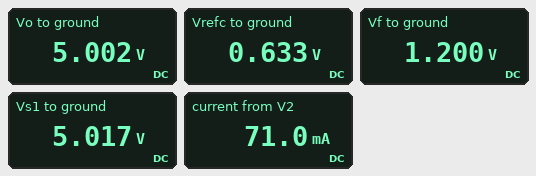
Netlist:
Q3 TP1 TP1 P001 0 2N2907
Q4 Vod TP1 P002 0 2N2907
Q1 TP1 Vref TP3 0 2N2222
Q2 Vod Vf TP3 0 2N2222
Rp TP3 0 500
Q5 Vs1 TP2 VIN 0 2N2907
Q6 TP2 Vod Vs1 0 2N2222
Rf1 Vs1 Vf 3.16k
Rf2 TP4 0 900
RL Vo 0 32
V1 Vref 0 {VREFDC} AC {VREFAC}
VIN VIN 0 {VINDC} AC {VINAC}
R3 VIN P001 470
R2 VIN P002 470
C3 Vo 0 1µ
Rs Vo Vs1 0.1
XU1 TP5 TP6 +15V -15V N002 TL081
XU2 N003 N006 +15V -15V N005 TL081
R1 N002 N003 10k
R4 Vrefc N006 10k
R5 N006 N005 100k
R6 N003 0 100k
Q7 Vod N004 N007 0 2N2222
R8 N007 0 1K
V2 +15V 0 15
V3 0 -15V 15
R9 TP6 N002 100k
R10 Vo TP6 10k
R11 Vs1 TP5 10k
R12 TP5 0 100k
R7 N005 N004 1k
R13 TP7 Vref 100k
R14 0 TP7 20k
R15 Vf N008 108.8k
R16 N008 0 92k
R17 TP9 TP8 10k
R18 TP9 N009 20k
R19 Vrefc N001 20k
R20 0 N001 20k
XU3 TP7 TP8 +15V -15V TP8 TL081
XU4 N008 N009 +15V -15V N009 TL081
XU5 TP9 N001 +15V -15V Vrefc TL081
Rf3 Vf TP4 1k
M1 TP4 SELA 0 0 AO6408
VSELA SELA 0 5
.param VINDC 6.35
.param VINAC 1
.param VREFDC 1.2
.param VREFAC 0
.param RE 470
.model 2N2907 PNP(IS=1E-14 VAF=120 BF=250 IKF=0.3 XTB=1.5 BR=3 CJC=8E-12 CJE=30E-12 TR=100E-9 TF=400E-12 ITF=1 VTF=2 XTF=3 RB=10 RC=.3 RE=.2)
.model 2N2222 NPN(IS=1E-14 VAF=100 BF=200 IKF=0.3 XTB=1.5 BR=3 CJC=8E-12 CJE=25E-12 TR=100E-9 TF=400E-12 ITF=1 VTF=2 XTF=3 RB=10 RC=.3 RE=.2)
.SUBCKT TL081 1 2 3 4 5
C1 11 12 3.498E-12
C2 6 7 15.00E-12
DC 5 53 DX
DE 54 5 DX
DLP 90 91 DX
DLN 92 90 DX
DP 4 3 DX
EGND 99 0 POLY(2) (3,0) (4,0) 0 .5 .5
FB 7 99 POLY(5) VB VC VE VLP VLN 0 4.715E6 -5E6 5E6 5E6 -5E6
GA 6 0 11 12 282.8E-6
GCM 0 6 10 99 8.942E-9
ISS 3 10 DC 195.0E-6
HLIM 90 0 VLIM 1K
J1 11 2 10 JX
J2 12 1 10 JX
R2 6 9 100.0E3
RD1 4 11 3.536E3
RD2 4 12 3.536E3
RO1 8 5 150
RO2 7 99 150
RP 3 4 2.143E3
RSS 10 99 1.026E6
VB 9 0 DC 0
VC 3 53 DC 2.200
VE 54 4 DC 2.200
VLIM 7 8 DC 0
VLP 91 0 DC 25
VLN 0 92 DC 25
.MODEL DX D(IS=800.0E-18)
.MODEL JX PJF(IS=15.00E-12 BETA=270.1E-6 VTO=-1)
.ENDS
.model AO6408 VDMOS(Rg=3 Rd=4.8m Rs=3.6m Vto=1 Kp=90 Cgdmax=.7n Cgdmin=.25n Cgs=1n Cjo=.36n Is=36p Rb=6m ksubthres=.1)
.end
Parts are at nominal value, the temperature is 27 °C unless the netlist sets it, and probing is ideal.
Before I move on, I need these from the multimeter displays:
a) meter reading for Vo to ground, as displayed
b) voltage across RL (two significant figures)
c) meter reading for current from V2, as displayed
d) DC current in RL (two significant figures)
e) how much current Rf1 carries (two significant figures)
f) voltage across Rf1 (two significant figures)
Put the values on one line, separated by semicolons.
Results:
5.002 V; 5.0 V; 71.0 mA; 160 mA; 1.2 mA; 3.8 V
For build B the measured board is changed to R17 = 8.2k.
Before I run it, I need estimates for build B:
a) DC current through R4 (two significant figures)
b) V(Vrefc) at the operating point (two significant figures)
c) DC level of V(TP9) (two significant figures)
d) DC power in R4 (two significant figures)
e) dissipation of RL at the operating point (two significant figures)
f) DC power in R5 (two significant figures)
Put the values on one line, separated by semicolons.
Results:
46 µA; 600 mV; 300 mV; 21 µW; 780 mW; 210 µW
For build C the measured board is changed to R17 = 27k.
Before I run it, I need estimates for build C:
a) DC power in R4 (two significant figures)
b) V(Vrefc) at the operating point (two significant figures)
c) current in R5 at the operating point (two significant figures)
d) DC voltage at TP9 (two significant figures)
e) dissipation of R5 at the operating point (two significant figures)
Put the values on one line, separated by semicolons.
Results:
44 µW; 800 mV; 66 µA; 400 mV; 440 µW
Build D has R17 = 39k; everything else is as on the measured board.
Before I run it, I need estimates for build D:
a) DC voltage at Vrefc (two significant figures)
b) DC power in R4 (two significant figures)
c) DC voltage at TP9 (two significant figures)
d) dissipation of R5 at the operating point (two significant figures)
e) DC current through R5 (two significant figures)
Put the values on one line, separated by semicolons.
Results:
860 mV; 52 µW; 430 mV; 520 µW; 72 µA
